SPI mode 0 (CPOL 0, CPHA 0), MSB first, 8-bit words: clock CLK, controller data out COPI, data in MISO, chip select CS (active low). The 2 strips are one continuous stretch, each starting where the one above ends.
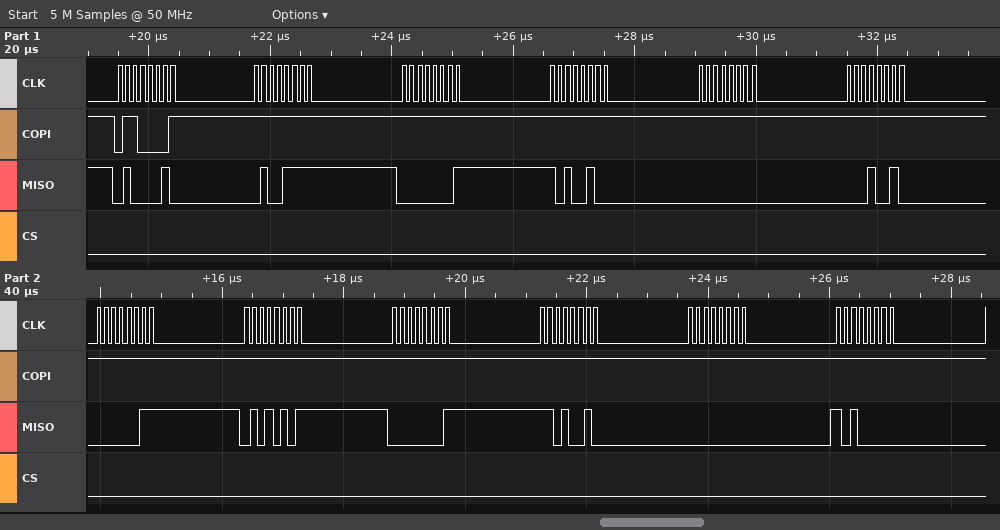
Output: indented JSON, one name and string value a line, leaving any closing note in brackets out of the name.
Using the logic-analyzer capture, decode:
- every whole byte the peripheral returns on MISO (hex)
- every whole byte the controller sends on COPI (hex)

{
  "every whole byte the peripheral returns on MISO": "42 4F 01 A4 00 12 03 55 01 D2 00 A0",
  "every whole byte the controller sends on COPI": "61 FF FF FF FF FF FF FF FF FF FF FF"
}
